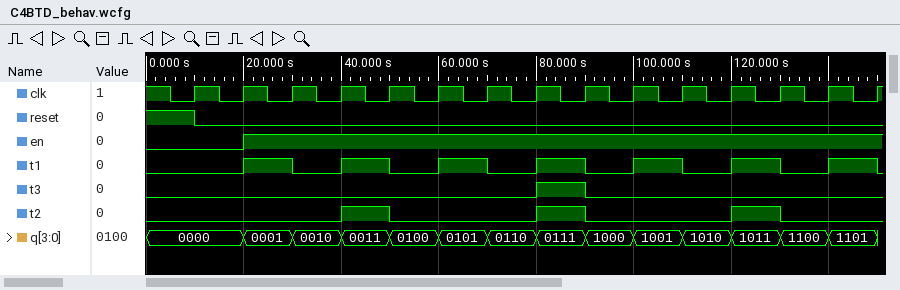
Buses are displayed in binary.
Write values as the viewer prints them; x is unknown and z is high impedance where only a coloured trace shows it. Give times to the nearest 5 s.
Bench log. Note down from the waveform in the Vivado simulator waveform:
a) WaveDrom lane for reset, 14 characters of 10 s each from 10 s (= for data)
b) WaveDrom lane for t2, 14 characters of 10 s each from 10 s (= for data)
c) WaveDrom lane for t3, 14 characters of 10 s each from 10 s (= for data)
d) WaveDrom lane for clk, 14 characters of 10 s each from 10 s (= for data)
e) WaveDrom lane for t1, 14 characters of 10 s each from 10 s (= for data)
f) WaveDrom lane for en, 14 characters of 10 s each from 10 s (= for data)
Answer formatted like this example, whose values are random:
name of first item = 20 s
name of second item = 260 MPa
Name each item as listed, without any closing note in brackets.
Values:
WaveDrom lane for reset, 14 characters of 10 s each from 10 s = {name: 'reset', wave: '0.............'}
WaveDrom lane for t2, 14 characters of 10 s each from 10 s = {name: 't2', wave: '0..10..10..10.'}
WaveDrom lane for t3, 14 characters of 10 s each from 10 s = {name: 't3', wave: '0......10.....'}
WaveDrom lane for clk, 14 characters of 10 s each from 10 s = {name: 'clk', wave: 'p.............'}
WaveDrom lane for t1, 14 characters of 10 s each from 10 s = {name: 't1', wave: '01010101010101'}
WaveDrom lane for en, 14 characters of 10 s each from 10 s = {name: 'en', wave: '01............'}
